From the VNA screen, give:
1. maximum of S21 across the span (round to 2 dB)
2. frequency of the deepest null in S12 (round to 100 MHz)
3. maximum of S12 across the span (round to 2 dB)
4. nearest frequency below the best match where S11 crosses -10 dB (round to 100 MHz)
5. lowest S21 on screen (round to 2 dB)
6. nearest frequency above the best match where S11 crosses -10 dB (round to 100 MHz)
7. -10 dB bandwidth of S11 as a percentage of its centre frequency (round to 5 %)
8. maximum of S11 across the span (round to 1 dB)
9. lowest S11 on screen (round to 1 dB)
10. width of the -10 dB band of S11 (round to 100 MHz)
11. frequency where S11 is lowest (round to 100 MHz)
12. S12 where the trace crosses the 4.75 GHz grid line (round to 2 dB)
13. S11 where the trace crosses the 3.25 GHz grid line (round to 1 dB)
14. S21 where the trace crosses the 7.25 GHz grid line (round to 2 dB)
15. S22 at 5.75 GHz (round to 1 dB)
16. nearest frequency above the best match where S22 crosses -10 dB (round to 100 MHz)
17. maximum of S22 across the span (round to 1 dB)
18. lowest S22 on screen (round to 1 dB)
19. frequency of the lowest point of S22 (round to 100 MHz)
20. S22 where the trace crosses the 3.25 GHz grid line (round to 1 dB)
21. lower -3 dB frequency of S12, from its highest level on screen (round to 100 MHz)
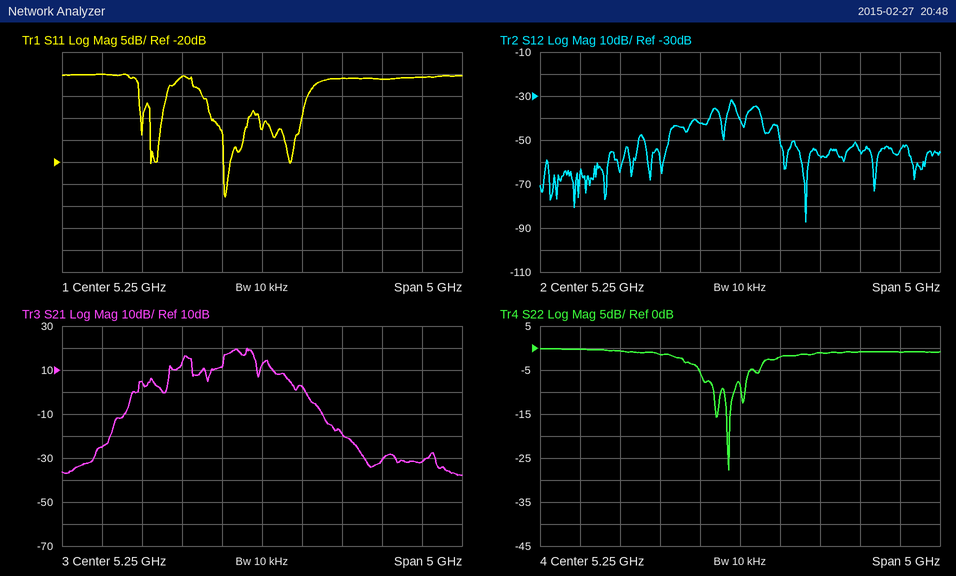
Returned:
20 dB
6.1 GHz
-32 dB
4.6 GHz
-38 dB
5.1 GHz
10 %
0 dB
-28 dB
500 MHz
4.8 GHz
-42 dB
0 dB
-32 dB
-2 dB
5.2 GHz
0 dB
-28 dB
5.1 GHz
0 dB
5.1 GHz
